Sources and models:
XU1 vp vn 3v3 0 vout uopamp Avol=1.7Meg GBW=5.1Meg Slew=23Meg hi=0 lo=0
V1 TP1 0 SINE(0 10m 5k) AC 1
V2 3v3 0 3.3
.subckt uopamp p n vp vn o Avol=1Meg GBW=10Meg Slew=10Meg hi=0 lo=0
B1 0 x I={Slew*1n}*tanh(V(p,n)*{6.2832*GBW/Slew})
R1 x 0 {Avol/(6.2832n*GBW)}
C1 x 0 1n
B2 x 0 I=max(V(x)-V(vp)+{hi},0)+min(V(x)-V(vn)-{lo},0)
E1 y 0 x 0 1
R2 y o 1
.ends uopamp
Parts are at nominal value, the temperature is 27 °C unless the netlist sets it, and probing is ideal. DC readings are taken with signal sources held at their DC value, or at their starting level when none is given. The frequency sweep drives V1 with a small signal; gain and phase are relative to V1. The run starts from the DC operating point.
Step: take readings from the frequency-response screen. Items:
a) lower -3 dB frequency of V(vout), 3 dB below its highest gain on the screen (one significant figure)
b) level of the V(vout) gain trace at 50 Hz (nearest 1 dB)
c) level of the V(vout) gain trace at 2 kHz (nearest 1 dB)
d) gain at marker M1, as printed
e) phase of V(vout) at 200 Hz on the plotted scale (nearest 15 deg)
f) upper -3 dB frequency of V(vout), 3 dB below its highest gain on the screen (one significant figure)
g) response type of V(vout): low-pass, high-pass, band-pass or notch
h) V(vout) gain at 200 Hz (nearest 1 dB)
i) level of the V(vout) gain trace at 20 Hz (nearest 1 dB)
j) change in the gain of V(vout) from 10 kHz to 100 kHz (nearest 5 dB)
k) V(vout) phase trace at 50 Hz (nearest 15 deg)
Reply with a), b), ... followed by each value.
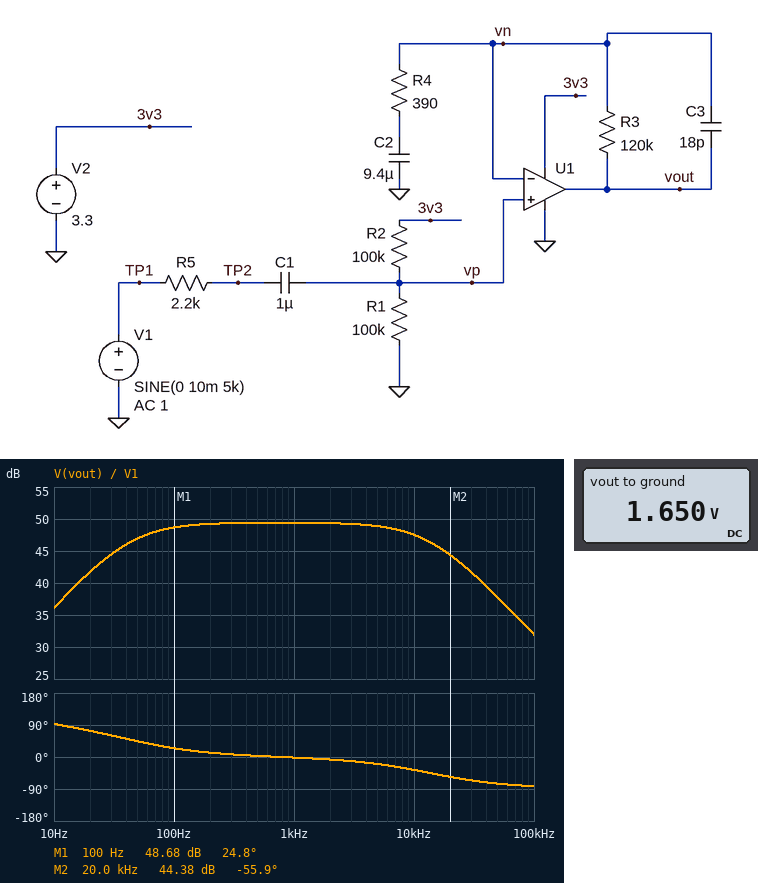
a) 40 Hz
b) 47 dB
c) 49 dB
d) 48.68 dB
e) 15 deg
f) 10 kHz
g) band-pass
h) 49 dB
i) 42 dB
j) -15 dB
k) 45 deg
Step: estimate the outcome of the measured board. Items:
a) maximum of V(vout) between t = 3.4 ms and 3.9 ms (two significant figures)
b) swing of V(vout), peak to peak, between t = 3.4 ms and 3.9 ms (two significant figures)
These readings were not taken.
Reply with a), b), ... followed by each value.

a) 3.3 V
b) 3.3 V
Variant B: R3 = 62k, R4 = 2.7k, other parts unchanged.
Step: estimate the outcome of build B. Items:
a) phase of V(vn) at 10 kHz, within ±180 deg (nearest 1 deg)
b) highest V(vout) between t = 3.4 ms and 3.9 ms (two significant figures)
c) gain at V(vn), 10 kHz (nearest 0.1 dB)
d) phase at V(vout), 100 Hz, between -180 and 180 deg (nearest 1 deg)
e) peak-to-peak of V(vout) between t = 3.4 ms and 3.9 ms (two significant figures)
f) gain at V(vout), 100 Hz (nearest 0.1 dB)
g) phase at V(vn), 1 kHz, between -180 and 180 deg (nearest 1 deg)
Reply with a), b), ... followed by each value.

a) -3 deg
b) 1.9 V
c) -0.4 dB
d) 5 deg
e) 460 mV
f) 27.2 dB
g) 0 deg
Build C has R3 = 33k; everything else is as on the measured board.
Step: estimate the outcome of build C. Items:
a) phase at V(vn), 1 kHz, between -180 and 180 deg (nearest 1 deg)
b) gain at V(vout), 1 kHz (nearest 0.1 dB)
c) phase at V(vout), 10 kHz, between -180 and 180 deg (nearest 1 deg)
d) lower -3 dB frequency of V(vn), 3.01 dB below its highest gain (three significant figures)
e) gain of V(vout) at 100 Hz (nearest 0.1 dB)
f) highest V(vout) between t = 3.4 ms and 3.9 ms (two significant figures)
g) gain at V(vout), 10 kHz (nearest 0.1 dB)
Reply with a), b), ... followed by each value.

a) -1 deg
b) 38.3 dB
c) -11 deg
d) 3.05 Hz
e) 37.5 dB
f) 2.5 V
g) 38.1 dB
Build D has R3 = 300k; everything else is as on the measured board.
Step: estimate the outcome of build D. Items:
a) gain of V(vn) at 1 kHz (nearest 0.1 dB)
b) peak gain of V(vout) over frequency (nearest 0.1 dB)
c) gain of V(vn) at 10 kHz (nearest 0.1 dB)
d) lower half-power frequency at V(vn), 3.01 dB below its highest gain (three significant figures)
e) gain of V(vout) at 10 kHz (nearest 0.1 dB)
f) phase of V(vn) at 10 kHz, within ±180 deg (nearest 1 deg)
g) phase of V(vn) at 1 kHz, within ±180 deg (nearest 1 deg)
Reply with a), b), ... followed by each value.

a) -0.5 dB
b) 57.3 dB
c) -6.3 dB
d) 3.08 Hz
e) 50.9 dB
f) -43 deg
g) -8 deg
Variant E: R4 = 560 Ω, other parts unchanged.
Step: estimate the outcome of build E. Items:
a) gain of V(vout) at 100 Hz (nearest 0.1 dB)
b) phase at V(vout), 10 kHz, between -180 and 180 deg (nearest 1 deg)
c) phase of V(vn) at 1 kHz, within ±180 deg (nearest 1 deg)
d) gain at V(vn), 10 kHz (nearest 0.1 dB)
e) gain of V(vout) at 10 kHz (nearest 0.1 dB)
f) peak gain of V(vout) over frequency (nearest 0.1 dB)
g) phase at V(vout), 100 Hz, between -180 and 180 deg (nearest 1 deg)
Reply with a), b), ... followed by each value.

a) 45.9 dB
b) -29 deg
c) -2 deg
d) -1.5 dB
e) 45.1 dB
f) 46.3 dB
g) 18 deg
